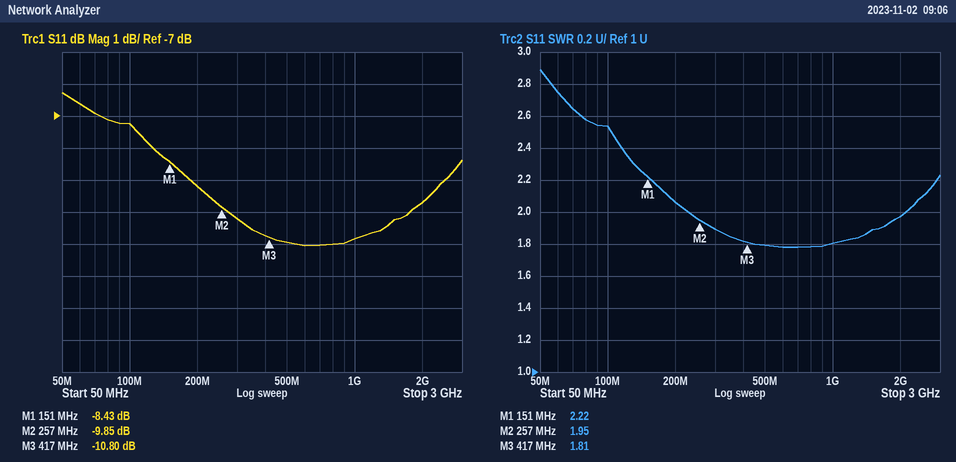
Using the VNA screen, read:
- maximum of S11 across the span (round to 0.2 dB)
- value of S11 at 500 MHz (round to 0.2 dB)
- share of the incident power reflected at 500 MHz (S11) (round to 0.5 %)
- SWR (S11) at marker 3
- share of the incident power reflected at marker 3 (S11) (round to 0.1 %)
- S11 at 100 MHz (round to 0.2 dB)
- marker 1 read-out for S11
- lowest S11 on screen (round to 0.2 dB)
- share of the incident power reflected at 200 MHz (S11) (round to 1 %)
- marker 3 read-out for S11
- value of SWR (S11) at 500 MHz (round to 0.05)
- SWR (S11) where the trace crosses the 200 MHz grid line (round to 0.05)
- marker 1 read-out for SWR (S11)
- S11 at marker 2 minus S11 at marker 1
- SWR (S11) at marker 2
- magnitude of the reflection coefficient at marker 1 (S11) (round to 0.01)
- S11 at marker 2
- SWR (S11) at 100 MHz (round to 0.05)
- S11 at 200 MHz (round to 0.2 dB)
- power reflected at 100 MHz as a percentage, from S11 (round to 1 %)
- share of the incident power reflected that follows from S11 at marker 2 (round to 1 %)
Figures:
-6.2 dB
-11.0 dB
8.0 %
1.81
8.3 %
-7.2 dB
-8.43 dB
-11.0 dB
12 %
-10.80 dB
1.80
2.05
2.22
-1.42 dB
1.95
0.38
-9.85 dB
2.55
-9.2 dB
19 %
10 %
